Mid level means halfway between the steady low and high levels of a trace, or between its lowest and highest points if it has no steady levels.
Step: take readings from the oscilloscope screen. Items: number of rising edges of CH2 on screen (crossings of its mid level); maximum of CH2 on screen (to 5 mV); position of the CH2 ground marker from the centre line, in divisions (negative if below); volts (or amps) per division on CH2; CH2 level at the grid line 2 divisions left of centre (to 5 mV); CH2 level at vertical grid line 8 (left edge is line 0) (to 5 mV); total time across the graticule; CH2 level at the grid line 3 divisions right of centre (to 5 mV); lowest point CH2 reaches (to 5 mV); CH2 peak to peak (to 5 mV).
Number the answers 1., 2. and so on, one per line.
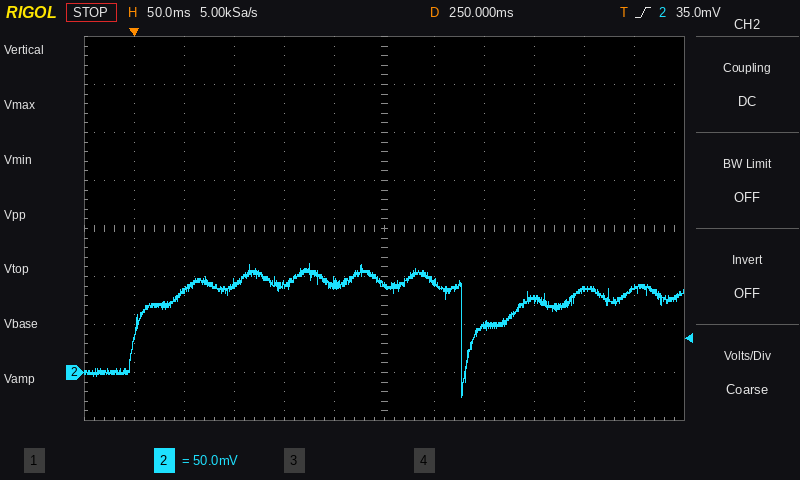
1. 2
2. 115 mV
3. -3.0 div
4. 50 mV
5. 90 mV
6. 50 mV
7. 600 ms
8. 75 mV
9. -25 mV
10. 140 mV
